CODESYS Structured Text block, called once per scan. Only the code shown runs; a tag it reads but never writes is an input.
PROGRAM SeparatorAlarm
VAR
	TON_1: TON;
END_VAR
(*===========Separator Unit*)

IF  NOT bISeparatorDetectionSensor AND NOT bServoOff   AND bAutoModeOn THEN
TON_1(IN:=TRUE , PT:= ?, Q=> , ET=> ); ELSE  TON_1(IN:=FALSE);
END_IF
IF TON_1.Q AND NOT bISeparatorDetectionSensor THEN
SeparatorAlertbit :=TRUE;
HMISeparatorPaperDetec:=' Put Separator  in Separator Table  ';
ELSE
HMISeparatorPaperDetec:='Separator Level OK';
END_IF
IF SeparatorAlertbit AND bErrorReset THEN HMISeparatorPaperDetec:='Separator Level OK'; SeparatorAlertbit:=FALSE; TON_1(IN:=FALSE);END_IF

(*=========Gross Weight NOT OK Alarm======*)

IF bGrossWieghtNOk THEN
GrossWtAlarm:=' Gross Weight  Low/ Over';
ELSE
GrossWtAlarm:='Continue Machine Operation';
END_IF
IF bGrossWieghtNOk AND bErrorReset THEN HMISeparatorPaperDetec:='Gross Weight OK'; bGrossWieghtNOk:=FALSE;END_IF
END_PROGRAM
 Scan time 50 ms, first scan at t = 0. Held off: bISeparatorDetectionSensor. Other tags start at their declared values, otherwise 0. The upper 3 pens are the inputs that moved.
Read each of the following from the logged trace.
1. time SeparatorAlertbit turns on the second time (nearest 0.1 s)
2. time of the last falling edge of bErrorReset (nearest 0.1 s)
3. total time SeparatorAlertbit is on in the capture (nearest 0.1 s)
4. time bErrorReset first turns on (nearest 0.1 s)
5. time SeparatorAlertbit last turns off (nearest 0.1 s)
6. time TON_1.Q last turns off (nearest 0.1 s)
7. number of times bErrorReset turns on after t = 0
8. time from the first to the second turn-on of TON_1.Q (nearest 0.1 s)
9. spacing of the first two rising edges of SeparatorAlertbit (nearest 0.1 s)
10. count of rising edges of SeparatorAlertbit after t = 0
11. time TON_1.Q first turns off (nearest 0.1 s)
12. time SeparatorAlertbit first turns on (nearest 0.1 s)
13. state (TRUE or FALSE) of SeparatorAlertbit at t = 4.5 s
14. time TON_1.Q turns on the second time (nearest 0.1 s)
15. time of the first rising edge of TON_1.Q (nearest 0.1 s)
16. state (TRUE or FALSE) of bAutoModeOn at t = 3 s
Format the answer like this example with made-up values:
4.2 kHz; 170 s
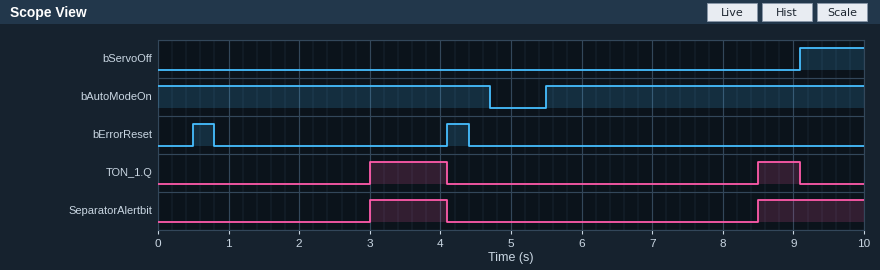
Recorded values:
8.5 s; 4.4 s; 2.6 s; 0.5 s; 4.1 s; 9.1 s; 2; 5.5 s; 5.5 s; 2; 4.1 s; 3.0 s; FALSE; 8.5 s; 3.0 s; TRUE
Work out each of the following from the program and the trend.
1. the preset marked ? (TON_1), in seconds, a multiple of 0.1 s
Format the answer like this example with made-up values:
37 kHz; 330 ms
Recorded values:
3.0 s
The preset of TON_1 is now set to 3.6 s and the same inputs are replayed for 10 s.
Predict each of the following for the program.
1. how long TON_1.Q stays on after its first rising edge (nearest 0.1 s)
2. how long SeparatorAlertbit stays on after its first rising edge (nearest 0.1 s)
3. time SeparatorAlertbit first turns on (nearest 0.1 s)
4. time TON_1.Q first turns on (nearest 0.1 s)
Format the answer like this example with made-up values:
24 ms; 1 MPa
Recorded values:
0.5 s; 0.5 s; 3.6 s; 3.6 s
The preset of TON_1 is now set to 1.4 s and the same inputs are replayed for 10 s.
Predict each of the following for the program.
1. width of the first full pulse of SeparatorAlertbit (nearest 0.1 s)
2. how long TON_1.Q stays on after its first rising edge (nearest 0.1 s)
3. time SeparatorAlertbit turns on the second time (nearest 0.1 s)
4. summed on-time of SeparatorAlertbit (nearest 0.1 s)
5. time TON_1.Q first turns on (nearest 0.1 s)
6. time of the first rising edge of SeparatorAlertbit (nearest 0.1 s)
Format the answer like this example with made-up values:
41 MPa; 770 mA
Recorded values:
2.7 s; 2.7 s; 6.9 s; 5.8 s; 1.4 s; 1.4 s
